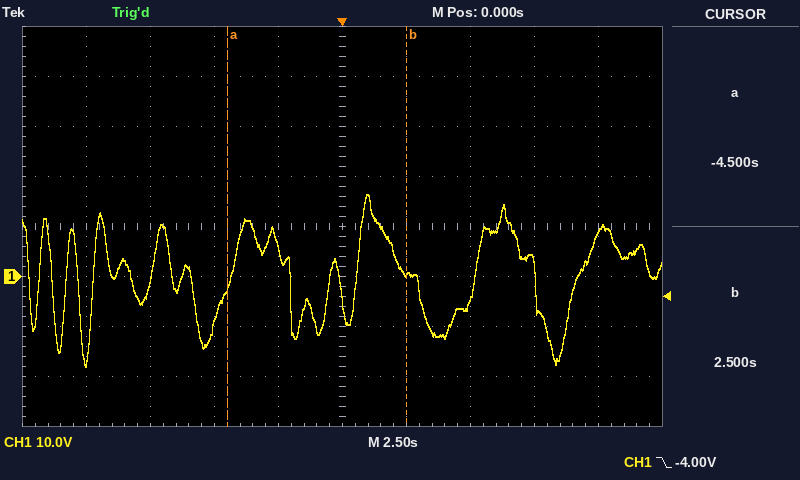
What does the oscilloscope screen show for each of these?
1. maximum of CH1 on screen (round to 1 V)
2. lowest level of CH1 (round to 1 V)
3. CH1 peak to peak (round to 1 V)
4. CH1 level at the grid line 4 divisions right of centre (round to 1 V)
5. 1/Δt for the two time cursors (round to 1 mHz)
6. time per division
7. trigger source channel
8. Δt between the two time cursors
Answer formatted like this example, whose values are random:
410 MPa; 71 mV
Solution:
16 V; -18 V; 34 V; 9 V; 143 mHz; 2.5 s; CH1; 7.00 s
